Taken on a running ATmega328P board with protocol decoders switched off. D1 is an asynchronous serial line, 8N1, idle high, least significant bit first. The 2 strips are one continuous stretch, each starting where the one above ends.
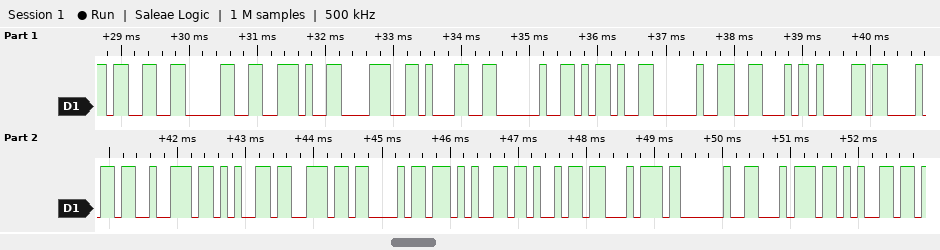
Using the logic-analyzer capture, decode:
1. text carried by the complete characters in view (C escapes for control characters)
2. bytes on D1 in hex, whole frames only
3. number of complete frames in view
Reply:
"30.81 - Fahrenheit te"
33 30 2E 38 31 20 2D 20 46 61 68 72 65 6E 68 65 69 74 20 74 65
21
